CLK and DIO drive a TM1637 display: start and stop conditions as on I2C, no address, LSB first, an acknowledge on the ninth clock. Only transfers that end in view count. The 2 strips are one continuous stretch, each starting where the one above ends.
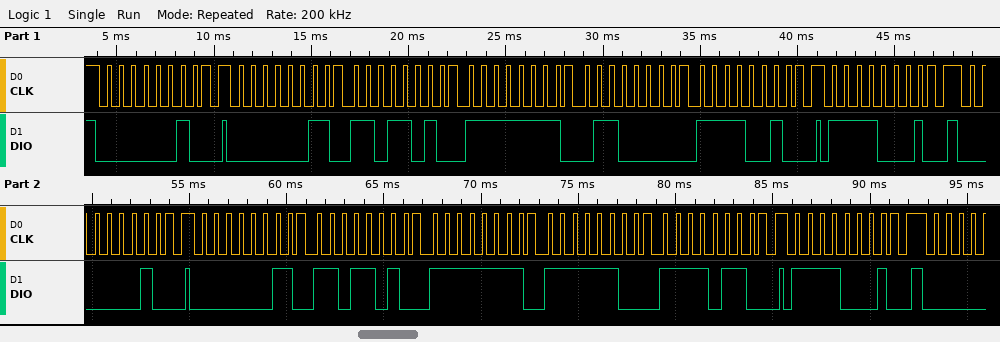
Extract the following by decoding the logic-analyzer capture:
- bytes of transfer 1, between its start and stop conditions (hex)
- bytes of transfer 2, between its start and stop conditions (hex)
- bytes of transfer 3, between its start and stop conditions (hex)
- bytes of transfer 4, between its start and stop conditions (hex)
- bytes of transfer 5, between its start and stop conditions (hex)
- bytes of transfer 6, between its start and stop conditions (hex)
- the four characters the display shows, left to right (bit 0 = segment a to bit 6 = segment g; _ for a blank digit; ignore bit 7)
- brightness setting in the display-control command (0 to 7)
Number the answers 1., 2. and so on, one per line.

1. 40
2. C0 5B FF 06 4F
3. 8F
4. 40
5. C0 5B FF 3F 6F
6. 8F
7. 2809
8. 7
